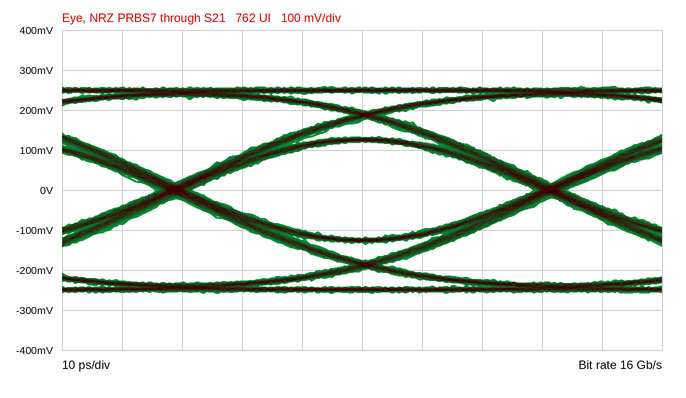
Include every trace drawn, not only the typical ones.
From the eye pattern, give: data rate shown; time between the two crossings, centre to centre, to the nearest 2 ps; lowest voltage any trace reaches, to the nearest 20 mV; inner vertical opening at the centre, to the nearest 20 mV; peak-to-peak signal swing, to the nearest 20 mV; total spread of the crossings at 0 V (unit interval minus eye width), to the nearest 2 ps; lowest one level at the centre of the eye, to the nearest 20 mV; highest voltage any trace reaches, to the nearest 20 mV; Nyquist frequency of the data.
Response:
16 Gb/s
62 ps
-260 mV
240 mV
520 mV
6 ps
120 mV
260 mV
8 GHz
